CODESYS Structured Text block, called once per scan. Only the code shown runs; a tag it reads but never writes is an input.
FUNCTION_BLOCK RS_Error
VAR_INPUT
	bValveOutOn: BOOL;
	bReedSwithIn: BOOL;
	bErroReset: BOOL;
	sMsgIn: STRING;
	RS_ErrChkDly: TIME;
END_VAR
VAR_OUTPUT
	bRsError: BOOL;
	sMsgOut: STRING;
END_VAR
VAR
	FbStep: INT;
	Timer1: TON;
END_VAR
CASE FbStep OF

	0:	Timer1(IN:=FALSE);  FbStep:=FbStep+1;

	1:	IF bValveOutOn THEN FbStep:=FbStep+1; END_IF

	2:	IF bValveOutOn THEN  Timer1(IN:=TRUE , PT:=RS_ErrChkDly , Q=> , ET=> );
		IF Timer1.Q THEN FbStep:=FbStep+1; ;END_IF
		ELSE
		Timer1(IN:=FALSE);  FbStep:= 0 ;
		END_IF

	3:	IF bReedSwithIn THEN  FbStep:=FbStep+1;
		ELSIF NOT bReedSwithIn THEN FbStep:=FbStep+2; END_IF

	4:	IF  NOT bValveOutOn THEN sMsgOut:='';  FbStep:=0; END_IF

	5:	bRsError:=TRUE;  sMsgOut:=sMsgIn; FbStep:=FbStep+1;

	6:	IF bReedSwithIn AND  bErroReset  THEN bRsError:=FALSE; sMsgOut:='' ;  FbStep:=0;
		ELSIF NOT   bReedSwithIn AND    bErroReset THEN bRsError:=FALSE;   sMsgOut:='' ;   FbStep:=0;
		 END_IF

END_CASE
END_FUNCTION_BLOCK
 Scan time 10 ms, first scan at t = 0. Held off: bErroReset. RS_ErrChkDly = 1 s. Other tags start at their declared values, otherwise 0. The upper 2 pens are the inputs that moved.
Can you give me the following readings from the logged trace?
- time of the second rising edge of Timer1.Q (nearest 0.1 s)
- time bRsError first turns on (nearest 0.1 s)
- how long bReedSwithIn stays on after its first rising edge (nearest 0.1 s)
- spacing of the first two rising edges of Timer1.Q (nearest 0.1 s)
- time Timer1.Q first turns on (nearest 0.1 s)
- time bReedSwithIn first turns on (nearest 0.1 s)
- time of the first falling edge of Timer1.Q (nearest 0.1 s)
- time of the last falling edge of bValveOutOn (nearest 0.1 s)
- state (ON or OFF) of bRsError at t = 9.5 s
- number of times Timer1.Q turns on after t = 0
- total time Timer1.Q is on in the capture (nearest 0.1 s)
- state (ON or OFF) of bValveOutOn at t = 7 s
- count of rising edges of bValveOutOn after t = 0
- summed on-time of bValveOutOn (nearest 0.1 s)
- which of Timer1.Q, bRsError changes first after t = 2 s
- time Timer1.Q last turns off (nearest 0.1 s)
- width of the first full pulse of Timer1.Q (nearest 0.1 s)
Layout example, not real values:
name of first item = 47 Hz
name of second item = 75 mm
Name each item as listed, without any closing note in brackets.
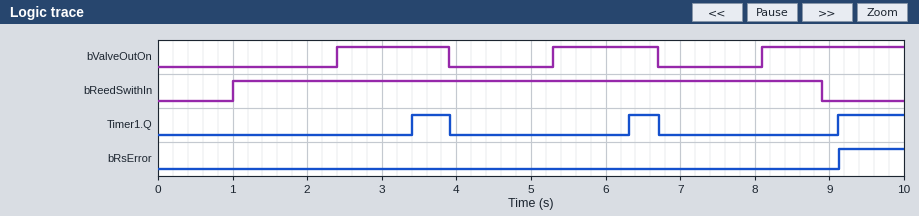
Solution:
time of the second rising edge of Timer1.Q = 6.3 s
time bRsError first turns on = 9.1 s
how long bReedSwithIn stays on after its first rising edge = 7.9 s
spacing of the first two rising edges of Timer1.Q = 2.9 s
time Timer1.Q first turns on = 3.4 s
time bReedSwithIn first turns on = 1.0 s
time of the first falling edge of Timer1.Q = 3.9 s
time of the last falling edge of bValveOutOn = 6.7 s
state (ON or OFF) of bRsError at t = 9.5 s = ON
number of times Timer1.Q turns on after t = 0 = 3
total time Timer1.Q is on in the capture = 1.8 s
state (ON or OFF) of bValveOutOn at t = 7 s = OFF
count of rising edges of bValveOutOn after t = 0 = 3
summed on-time of bValveOutOn = 4.8 s
which of Timer1.Q, bRsError changes first after t = 2 s = Timer1.Q
time Timer1.Q last turns off = 6.7 s
width of the first full pulse of Timer1.Q = 0.5 s
